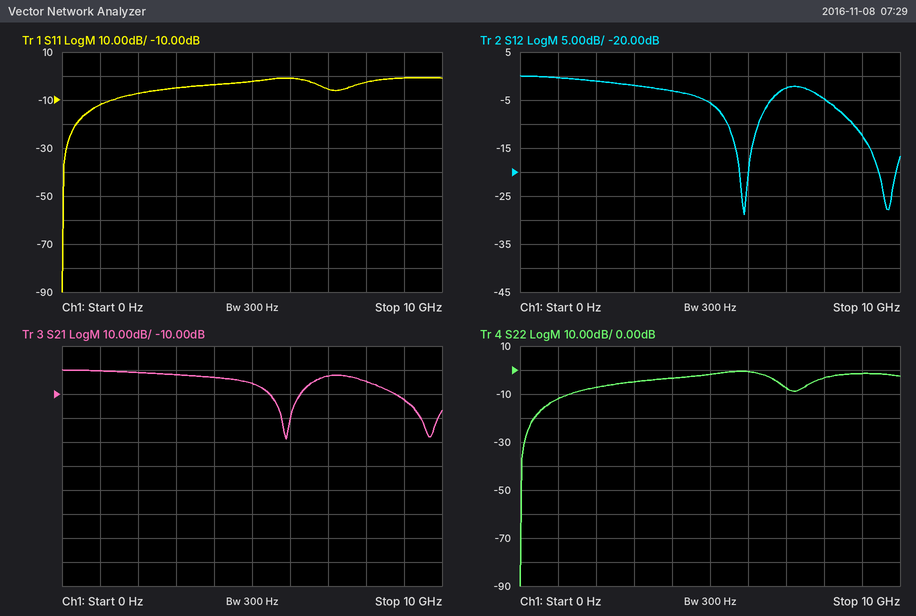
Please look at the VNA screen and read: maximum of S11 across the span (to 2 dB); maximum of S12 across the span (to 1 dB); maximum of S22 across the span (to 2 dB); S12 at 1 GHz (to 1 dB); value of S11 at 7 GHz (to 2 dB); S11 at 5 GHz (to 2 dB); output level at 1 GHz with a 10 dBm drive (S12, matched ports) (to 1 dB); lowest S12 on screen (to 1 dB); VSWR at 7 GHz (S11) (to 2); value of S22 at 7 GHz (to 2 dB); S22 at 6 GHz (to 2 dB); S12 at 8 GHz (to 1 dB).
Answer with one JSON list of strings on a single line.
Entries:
["0 dB", "0 dB", "0 dB", "0 dB", "-6 dB", "-2 dB", "10 dBm", "-29 dB", "4", "-8 dB", "0 dB", "-5 dB"]
